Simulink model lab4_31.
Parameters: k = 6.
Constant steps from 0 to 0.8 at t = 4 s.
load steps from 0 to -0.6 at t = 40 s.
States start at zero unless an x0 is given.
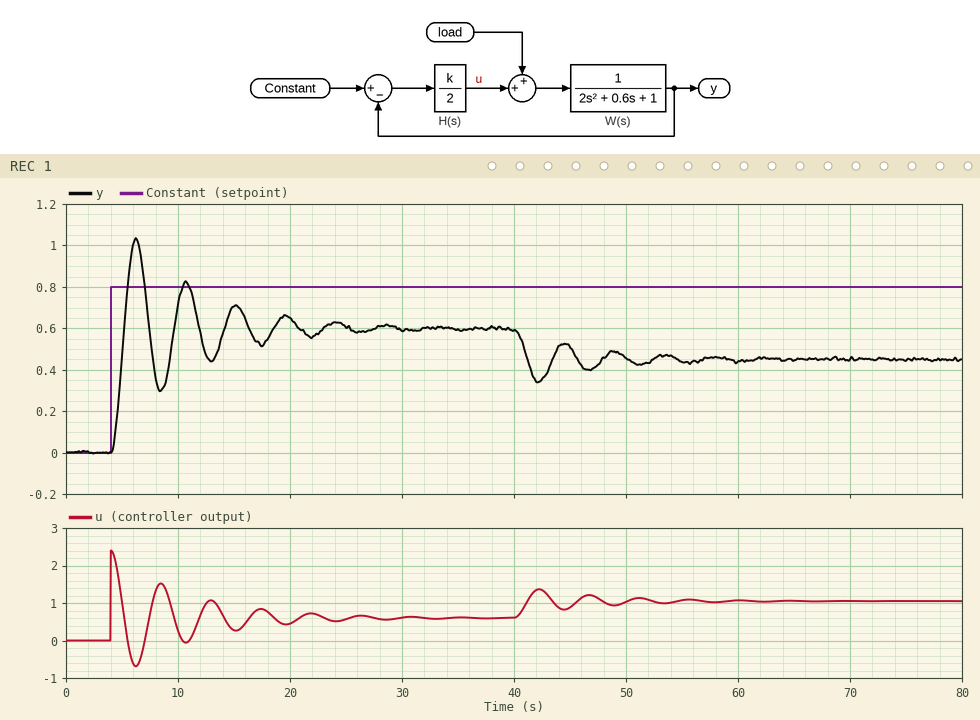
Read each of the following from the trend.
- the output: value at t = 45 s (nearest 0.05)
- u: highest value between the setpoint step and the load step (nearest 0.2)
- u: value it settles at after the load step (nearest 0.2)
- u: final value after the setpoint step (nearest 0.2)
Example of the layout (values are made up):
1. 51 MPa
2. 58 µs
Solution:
1. 0.50
2. 2.4
3. 1.0
4. 0.6
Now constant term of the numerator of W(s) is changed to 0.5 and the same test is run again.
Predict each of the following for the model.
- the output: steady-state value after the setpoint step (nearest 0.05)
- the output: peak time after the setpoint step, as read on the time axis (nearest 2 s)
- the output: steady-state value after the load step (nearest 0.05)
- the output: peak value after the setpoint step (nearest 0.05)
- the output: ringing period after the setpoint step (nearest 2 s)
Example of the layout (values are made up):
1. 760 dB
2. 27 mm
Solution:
1. 0.50
2. 6 s
3. 0.35
4. 0.80
5. 6 s
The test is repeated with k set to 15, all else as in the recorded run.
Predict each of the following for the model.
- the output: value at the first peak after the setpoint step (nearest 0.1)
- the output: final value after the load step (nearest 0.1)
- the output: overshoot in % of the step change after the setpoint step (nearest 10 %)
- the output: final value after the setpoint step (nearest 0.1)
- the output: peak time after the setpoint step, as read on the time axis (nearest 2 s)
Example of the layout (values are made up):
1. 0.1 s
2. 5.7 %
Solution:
1. 1.3
2. 0.6
3. 80 %
4. 0.7
5. 6 s
